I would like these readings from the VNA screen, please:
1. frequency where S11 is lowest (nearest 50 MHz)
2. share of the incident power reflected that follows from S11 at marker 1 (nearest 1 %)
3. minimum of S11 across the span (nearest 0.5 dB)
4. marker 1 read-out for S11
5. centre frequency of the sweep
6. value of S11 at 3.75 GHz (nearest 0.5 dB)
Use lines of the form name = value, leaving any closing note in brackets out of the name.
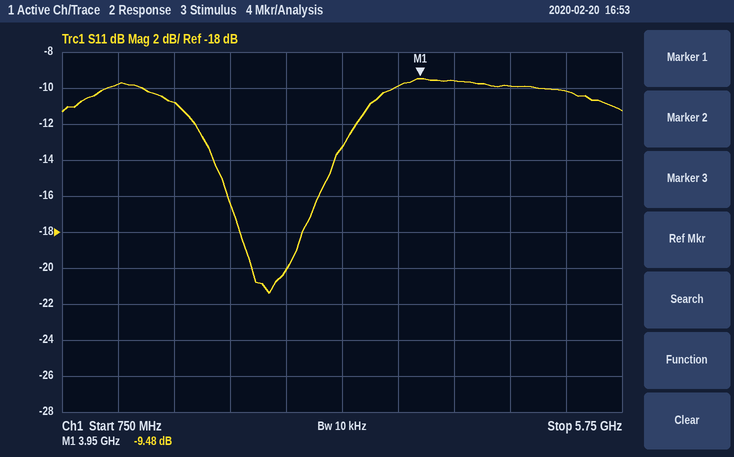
frequency where S11 is lowest = 2.60 GHz
share of the incident power reflected that follows from S11 at marker 1 = 11 %
minimum of S11 across the span = -21.5 dB
marker 1 read-out for S11 = -9.48 dB
centre frequency of the sweep = 3.25 GHz
value of S11 at 3.75 GHz = -10.0 dB
